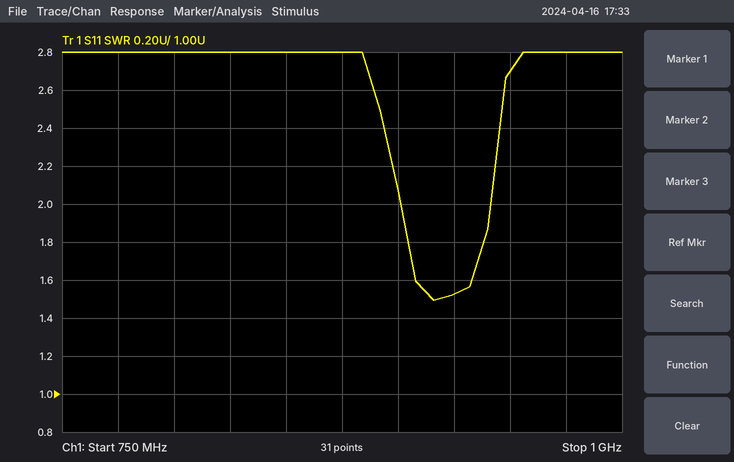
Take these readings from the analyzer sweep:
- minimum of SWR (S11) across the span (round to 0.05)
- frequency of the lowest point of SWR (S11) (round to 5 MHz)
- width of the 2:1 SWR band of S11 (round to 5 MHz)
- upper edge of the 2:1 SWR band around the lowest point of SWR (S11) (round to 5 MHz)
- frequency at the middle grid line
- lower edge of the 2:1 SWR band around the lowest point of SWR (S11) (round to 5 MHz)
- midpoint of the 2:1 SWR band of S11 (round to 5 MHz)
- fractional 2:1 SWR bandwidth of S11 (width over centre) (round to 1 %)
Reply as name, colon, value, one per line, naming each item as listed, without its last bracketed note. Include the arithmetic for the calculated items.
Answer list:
minimum of SWR (S11) across the span: 1.50
frequency of the lowest point of SWR (S11): 915 MHz
width of the 2:1 SWR band of S11: 940 MHz − 900 MHz = 40 MHz
upper edge of the 2:1 SWR band around the lowest point of SWR (S11): 940 MHz
frequency at the middle grid line: 875 MHz
lower edge of the 2:1 SWR band around the lowest point of SWR (S11): 900 MHz
midpoint of the 2:1 SWR band of S11: 920 MHz
fractional 2:1 SWR bandwidth of S11 (width over centre): 40 MHz / 920 MHz ≈ 4 %
